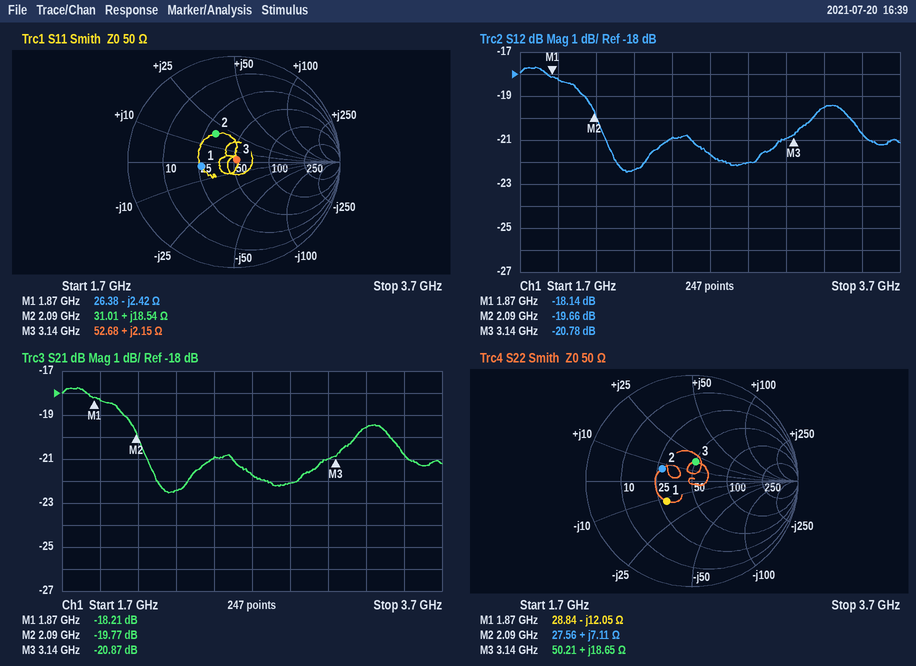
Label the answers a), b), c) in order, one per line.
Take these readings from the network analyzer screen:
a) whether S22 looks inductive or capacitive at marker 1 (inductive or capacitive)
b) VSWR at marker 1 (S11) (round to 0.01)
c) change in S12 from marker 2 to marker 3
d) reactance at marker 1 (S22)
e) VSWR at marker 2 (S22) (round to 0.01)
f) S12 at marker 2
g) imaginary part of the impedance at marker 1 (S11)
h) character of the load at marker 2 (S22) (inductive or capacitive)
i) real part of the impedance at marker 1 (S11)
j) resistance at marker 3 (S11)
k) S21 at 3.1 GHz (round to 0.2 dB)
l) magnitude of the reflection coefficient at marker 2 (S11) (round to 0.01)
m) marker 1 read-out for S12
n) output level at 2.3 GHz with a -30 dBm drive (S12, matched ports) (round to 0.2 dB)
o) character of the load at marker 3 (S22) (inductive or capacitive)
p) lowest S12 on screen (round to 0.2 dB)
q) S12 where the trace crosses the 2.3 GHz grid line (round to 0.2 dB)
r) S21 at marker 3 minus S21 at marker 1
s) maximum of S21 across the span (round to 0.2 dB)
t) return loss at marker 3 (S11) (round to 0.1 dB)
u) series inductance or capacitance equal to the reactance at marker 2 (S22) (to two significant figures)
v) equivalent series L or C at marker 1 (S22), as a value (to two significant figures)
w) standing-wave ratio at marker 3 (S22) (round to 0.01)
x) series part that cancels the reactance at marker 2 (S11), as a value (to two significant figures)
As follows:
a) capacitive
b) 1.90
c) -1.12 dB
d) -12.05 Ω
e) 1.87
f) -19.66 dB
g) -2.42 Ω
h) inductive
i) 26.38 Ω
j) 52.68 Ω
k) -21.0 dB
l) 0.32
m) -18.14 dB
n) -52.4 dBm
o) inductive
p) -22.4 dB
q) -22.4 dB
r) -2.66 dB
s) -17.8 dB
t) 29.5 dB
u) 540 pH
v) 7.1 pF
w) 1.45
x) 4.1 pF
